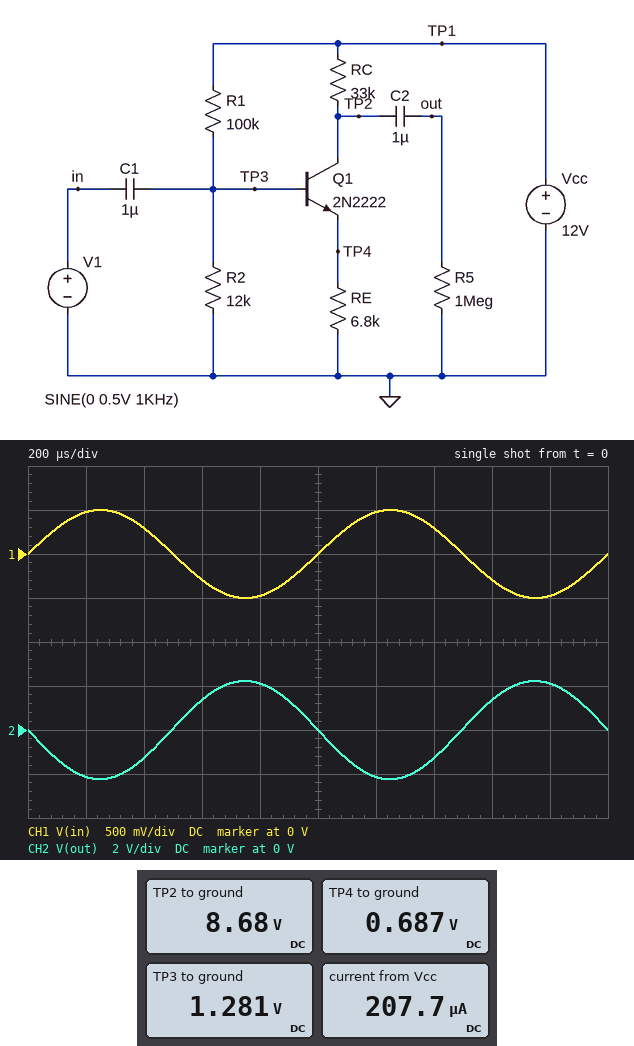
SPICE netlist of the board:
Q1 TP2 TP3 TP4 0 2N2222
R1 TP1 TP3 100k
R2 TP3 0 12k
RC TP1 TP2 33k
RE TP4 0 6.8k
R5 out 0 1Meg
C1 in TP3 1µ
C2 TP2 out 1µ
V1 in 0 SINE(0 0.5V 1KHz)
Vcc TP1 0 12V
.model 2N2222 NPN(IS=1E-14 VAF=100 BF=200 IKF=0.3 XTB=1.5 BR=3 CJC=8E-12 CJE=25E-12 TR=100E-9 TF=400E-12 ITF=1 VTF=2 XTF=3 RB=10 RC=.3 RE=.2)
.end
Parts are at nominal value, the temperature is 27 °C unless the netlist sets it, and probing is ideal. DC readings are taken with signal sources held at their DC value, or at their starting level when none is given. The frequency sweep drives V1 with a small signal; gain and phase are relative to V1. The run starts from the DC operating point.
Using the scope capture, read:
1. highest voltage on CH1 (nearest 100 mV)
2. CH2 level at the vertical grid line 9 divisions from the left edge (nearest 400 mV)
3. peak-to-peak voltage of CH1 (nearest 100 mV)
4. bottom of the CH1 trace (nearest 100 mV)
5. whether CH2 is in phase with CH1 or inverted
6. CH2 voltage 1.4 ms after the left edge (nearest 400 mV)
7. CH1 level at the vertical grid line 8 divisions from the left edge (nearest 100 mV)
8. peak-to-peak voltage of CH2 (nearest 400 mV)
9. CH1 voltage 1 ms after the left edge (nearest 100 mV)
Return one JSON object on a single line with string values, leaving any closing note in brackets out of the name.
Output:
{"highest voltage on CH1": "500 mV", "CH2 level at the vertical grid line 9 divisions from the left edge": "2.0 V", "peak-to-peak voltage of CH1": "1.0 V", "bottom of the CH1 trace": "-500 mV", "whether CH2 is in phase with CH1 or inverted": "inverted", "CH2 voltage 1.4 ms after the left edge": "-1.2 V", "CH1 level at the vertical grid line 8 divisions from the left edge": "-300 mV", "peak-to-peak voltage of CH2": "4.4 V", "CH1 voltage 1 ms after the left edge": "0 V"}
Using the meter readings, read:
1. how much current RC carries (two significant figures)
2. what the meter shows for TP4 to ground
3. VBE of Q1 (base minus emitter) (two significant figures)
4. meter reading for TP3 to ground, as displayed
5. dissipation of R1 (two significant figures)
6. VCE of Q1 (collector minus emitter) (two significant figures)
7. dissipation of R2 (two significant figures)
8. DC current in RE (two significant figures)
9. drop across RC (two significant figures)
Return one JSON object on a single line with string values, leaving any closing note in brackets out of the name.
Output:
{"how much current RC carries": "100 µA", "what the meter shows for TP4 to ground": "0.687 V", "VBE of Q1 (base minus emitter)": "590 mV", "meter reading for TP3 to ground, as displayed": "1.281 V", "dissipation of R1": "1.1 mW", "VCE of Q1 (collector minus emitter)": "8.0 V", "dissipation of R2": "140 µW", "DC current in RE": "100 µA", "drop across RC": "3.3 V"}
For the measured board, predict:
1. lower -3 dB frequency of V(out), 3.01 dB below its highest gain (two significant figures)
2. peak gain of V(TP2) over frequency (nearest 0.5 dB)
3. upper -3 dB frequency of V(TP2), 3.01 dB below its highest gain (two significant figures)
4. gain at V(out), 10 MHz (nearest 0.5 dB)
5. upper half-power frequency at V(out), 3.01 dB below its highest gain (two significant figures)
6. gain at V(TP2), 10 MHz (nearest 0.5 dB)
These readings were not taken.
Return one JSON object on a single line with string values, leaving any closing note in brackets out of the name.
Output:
{"lower -3 dB frequency of V(out), 3.01 dB below its highest gain": "15 Hz", "peak gain of V(TP2) over frequency": "13.0 dB", "upper -3 dB frequency of V(TP2), 3.01 dB below its highest gain": "1.5 MHz", "gain at V(out), 10 MHz": "2.5 dB", "upper half-power frequency at V(out), 3.01 dB below its highest gain": "1.5 MHz", "gain at V(TP2), 10 MHz": "2.5 dB"}
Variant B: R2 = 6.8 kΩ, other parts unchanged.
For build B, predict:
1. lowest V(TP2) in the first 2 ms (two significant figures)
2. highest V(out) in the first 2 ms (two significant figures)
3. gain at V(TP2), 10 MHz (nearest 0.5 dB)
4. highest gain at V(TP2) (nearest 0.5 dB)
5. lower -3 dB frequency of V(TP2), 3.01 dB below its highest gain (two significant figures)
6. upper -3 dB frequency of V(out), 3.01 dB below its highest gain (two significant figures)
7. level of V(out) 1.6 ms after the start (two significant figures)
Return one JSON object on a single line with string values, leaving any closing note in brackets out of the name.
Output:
{"lowest V(TP2) in the first 2 ms": "8.9 V", "highest V(out) in the first 2 ms": "940 mV", "gain at V(TP2), 10 MHz": "2.0 dB", "highest gain at V(TP2)": "12.5 dB", "lower -3 dB frequency of V(TP2), 3.01 dB below its highest gain": "25 Hz", "upper -3 dB frequency of V(out), 3.01 dB below its highest gain": "1.7 MHz", "level of V(out) 1.6 ms after the start": "930 mV"}
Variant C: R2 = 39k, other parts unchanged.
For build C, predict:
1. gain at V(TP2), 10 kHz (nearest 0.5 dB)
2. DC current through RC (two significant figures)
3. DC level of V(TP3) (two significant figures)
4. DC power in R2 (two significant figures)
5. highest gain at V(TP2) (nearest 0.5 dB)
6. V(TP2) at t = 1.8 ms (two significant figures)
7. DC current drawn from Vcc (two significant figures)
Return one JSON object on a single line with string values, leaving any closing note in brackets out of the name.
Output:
{"gain at V(TP2), 10 kHz": "-2.0 dB", "DC current through RC": "300 µA", "DC level of V(TP3)": "2.8 V", "DC power in R2": "200 µW", "highest gain at V(TP2)": "0 dB", "V(TP2) at t = 1.8 ms": "3.9 V", "DC current drawn from Vcc": "390 µA"}
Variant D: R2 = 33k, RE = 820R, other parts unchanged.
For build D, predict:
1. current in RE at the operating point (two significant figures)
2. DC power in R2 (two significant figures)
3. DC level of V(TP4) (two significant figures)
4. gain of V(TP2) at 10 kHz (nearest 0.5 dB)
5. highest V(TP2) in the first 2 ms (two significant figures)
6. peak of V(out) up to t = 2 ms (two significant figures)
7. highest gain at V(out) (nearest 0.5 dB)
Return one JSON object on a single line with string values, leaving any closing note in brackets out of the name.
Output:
{"current in RE at the operating point": "430 µA", "DC power in R2": "30 µW", "DC level of V(TP4)": "350 mV", "gain of V(TP2) at 10 kHz": "-4.0 dB", "highest V(TP2) in the first 2 ms": "12 V", "peak of V(out) up to t = 2 ms": "11 V", "highest gain at V(out)": "0 dB"}
